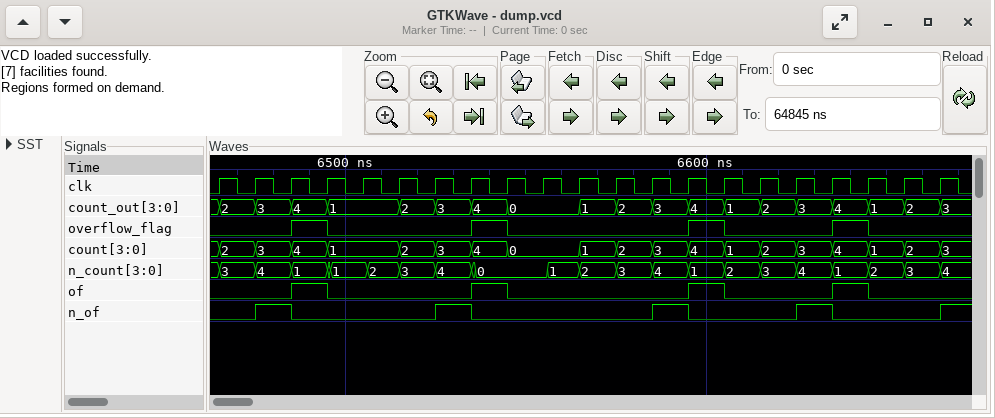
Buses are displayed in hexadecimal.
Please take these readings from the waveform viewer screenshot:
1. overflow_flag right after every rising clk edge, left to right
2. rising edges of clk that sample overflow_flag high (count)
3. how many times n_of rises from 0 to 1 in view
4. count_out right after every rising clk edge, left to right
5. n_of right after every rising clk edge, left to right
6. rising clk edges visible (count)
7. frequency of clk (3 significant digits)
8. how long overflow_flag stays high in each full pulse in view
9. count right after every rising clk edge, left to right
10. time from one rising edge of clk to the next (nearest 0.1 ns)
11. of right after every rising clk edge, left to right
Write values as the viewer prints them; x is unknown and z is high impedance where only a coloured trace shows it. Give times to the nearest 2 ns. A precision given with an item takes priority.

0 0 1 0 0 0 0 1 0 0 0 0 0 1 0 0 0 1 0 0 0
4
5
2, 3, 4, 1, 1, 2, 3, 4, 0, 0, 1, 2, 3, 4, 1, 2, 3, 4, 1, 2, 3
0 1 0 0 0 0 1 0 0 0 0 0 1 0 0 0 1 0 0 0 1
21
100 MHz
10 ns, 10 ns, 10 ns, 10 ns
2, 3, 4, 1, 1, 2, 3, 4, 0, 0, 1, 2, 3, 4, 1, 2, 3, 4, 1, 2, 3
10 ns
0 0 1 0 0 0 0 1 0 0 0 0 0 1 0 0 0 1 0 0 0
